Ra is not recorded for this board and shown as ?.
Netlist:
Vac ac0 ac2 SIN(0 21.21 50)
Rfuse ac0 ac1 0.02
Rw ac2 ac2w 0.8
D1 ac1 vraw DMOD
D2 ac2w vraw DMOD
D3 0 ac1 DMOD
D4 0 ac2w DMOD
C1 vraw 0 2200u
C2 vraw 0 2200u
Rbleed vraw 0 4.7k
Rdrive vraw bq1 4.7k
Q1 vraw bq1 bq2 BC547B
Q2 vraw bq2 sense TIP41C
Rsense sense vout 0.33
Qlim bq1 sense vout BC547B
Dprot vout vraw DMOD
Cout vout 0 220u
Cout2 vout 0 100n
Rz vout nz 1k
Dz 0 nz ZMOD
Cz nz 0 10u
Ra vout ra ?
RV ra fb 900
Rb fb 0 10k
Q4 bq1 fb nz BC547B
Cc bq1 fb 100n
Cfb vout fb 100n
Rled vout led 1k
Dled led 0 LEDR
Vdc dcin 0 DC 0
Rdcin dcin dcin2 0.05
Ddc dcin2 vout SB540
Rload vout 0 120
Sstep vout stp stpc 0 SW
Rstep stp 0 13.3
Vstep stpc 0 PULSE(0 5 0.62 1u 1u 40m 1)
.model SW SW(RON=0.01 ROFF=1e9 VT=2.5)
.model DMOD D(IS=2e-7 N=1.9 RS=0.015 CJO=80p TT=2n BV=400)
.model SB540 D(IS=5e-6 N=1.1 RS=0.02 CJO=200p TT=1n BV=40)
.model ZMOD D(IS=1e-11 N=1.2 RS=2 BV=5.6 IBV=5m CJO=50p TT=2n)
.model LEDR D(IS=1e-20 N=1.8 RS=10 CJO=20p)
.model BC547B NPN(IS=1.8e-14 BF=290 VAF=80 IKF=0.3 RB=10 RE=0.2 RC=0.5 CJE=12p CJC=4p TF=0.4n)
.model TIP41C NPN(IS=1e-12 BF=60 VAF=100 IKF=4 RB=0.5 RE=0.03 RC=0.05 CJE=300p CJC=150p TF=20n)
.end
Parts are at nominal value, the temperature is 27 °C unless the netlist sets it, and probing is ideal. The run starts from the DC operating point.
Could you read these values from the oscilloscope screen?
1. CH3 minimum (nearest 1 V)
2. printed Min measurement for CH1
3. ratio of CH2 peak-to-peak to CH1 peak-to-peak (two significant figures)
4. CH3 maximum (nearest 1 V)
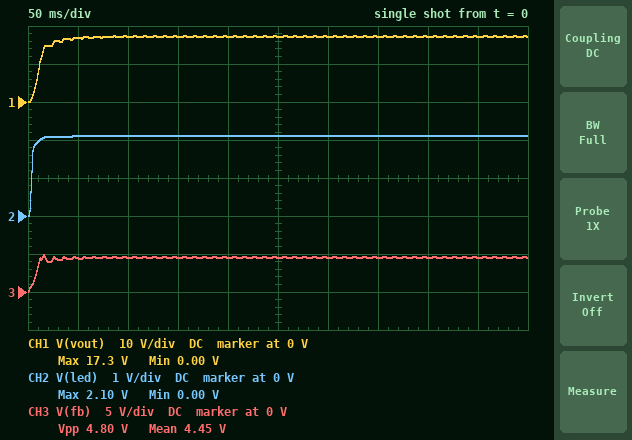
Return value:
0 V
0.00 V
0.12
5 V
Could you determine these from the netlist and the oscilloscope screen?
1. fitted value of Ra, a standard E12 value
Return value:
27 kΩ
